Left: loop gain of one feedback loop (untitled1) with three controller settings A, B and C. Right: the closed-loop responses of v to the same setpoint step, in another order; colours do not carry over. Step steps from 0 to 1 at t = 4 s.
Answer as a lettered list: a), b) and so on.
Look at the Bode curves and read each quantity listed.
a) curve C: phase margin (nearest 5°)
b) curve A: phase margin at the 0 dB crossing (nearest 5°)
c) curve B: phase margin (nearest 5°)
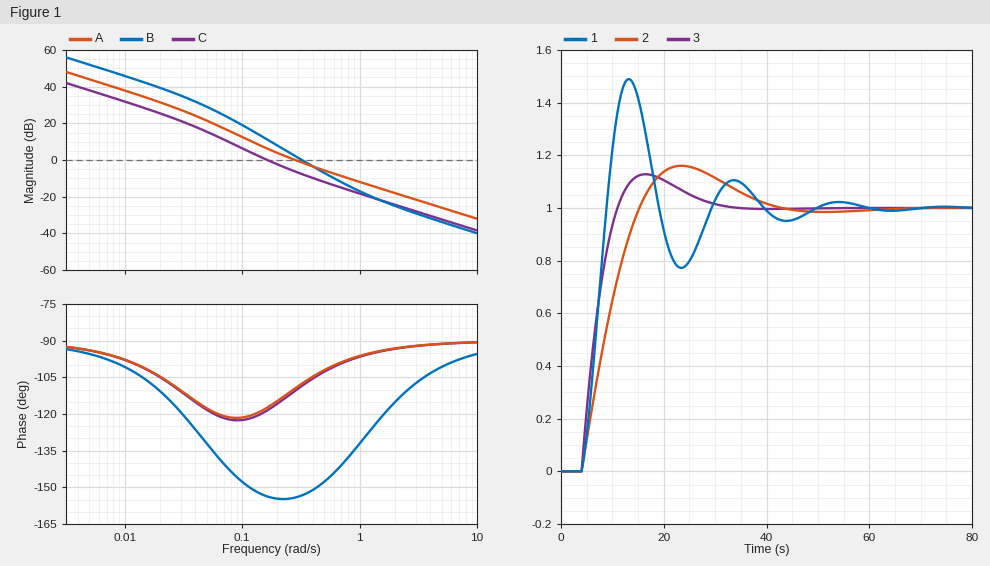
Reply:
a) 60°
b) 70°
c) 25°
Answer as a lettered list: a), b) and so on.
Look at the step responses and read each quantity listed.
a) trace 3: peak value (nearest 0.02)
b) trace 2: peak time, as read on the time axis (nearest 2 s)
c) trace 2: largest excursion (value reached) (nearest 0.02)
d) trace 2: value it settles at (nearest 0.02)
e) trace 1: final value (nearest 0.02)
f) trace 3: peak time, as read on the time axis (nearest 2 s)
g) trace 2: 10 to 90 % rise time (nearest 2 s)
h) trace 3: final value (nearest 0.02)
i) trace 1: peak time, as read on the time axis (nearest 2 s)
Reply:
a) 1.12
b) 24 s
c) 1.16
d) 1.00
e) 1.00
f) 16 s
g) 8 s
h) 1.00
i) 14 s
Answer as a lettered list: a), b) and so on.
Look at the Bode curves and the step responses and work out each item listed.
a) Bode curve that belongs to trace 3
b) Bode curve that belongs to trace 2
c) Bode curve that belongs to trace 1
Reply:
a) A
b) C
c) B
